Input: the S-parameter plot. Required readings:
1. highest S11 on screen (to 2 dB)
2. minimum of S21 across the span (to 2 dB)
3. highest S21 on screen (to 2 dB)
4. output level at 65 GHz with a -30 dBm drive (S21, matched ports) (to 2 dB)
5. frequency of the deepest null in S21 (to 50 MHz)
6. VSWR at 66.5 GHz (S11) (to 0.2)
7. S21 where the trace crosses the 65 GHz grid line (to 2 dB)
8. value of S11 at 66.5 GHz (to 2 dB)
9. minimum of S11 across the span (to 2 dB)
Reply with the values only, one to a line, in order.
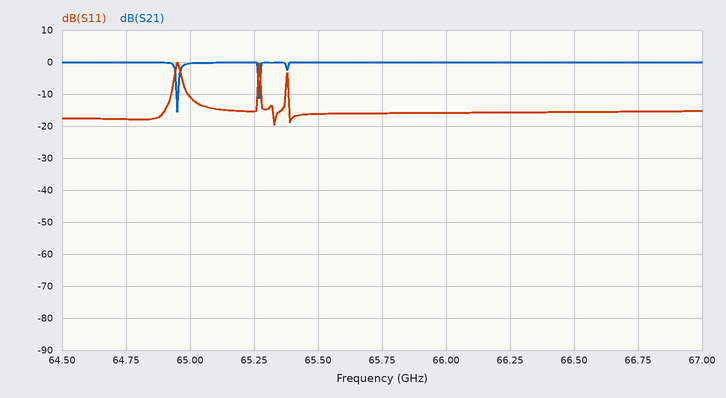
0 dB
-16 dB
0 dB
-30 dBm
64.95 GHz
1.4
0 dB
-16 dB
-20 dB
